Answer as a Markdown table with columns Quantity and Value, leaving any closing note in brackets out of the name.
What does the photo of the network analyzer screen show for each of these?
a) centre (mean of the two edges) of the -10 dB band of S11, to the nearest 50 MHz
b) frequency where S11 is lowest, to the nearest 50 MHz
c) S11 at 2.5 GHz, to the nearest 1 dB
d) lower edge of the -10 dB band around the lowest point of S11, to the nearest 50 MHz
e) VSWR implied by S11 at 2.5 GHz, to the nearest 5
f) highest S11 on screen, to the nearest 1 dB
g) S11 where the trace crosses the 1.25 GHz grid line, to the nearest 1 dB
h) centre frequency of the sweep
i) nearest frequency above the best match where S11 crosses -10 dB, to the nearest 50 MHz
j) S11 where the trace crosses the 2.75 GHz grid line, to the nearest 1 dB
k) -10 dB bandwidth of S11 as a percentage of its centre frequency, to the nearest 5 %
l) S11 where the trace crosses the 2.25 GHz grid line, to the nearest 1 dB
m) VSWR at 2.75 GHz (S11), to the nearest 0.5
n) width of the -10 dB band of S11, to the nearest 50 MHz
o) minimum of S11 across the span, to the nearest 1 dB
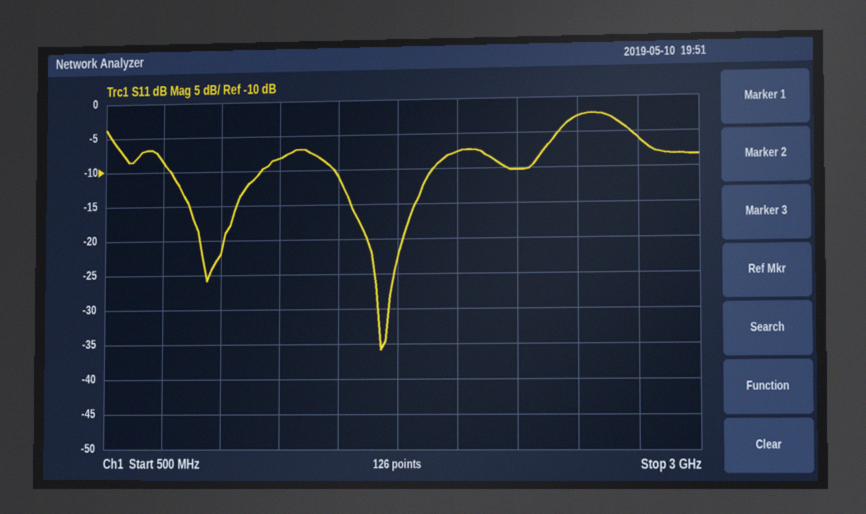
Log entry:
| Quantity | Value |
|---|---|
| centre (mean of the two edges) of the -10 dB band of S11, to the nearest 50 MHz | 1.70 GHz |
| frequency where S11 is lowest, to the nearest 50 MHz | 1.70 GHz |
| S11 at 2.5 GHz, to the nearest 1 dB | -3 dB |
| lower edge of the -10 dB band around the lowest point of S11, to the nearest 50 MHz | 1.50 GHz |
| VSWR implied by S11 at 2.5 GHz, to the nearest 5 | 5 |
| highest S11 on screen, to the nearest 1 dB | -2 dB |
| S11 where the trace crosses the 1.25 GHz grid line, to the nearest 1 dB | -8 dB |
| centre frequency of the sweep | 1.75 GHz |
| nearest frequency above the best match where S11 crosses -10 dB, to the nearest 50 MHz | 1.90 GHz |
| S11 where the trace crosses the 2.75 GHz grid line, to the nearest 1 dB | -6 dB |
| -10 dB bandwidth of S11 as a percentage of its centre frequency, to the nearest 5 % | 25 % |
| S11 where the trace crosses the 2.25 GHz grid line, to the nearest 1 dB | -10 dB |
| VSWR at 2.75 GHz (S11), to the nearest 0.5 | 3.0 |
| width of the -10 dB band of S11, to the nearest 50 MHz | 400 MHz |
| minimum of S11 across the span, to the nearest 1 dB | -36 dB |
